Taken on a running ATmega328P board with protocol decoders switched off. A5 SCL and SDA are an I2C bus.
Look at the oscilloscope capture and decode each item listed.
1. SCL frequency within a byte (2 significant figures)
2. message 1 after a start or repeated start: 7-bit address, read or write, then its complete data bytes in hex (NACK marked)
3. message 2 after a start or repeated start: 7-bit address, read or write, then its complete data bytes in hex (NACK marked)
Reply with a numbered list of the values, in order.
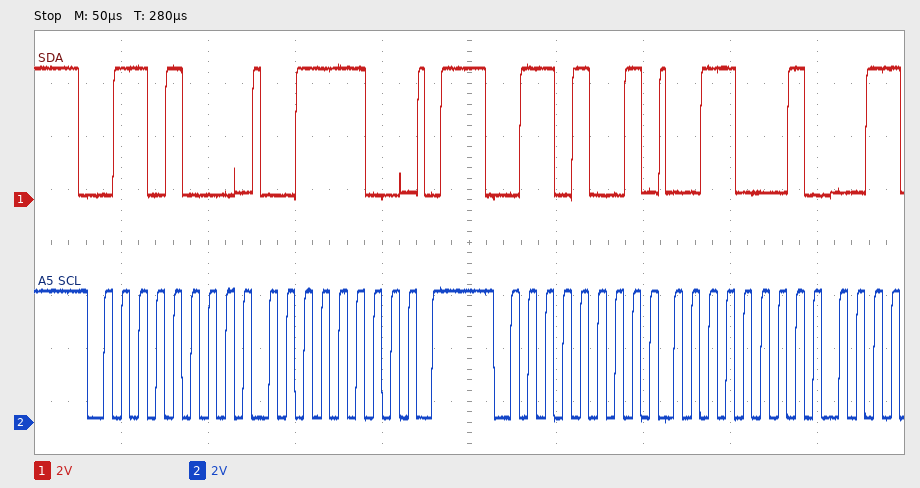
1. 100 kHz
2. 0x34 write: 3C
3. 0x34 read: 31
